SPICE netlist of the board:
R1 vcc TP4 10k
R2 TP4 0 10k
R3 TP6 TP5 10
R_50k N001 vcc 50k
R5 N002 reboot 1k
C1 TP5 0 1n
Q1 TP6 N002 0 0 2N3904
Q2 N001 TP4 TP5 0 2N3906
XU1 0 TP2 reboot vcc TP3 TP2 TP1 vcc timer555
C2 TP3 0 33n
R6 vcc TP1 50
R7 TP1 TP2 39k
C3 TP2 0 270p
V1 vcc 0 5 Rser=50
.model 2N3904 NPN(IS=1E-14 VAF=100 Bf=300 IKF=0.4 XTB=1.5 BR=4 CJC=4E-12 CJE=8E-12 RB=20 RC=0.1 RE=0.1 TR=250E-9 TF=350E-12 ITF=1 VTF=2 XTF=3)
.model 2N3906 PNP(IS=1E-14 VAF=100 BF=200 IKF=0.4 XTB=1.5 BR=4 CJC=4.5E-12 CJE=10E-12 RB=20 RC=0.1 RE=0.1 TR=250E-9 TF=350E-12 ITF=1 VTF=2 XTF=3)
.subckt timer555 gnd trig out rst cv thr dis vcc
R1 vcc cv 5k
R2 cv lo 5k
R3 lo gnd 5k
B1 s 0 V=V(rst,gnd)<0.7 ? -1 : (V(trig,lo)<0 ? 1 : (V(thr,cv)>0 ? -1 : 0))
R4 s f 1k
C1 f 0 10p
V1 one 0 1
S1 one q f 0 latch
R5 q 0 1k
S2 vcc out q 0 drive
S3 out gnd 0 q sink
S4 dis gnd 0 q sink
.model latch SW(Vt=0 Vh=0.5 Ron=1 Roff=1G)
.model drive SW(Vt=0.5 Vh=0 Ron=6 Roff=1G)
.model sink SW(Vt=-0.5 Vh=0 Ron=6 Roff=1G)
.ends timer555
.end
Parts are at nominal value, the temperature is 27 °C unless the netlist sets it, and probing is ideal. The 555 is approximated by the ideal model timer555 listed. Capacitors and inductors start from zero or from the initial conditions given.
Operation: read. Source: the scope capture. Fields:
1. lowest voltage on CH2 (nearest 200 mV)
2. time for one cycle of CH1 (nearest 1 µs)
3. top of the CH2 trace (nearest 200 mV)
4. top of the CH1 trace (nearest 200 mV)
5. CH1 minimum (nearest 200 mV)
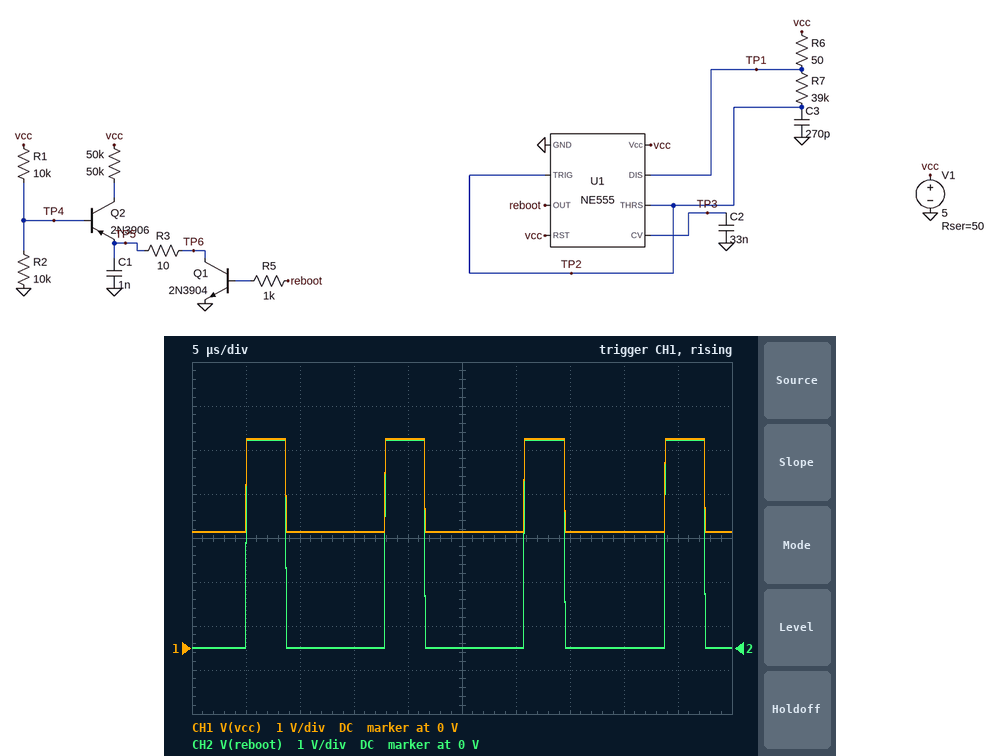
0 V
13 µs
4.8 V
4.8 V
2.6 V
